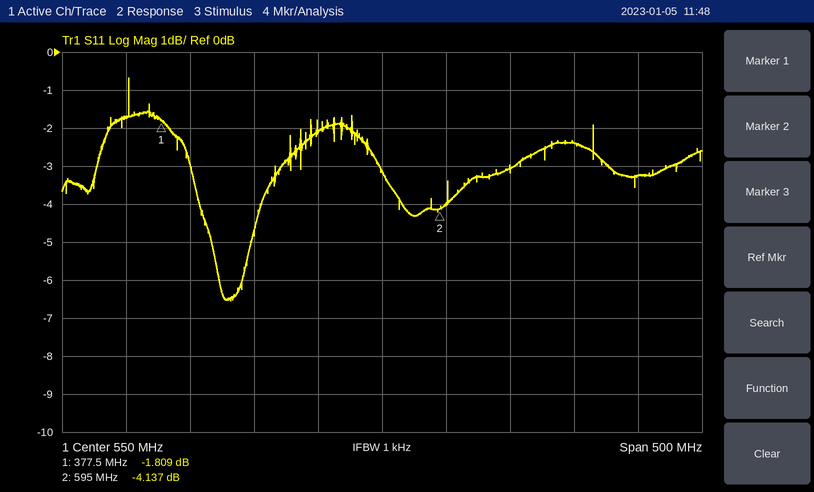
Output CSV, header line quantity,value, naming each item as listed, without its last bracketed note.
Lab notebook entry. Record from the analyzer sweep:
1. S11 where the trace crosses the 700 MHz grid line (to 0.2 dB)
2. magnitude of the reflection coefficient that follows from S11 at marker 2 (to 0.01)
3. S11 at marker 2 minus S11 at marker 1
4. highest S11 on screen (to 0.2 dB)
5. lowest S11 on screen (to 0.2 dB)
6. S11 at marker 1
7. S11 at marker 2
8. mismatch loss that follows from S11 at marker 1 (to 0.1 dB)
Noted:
quantity,value
S11 where the trace crosses the 700 MHz grid line,-2.4 dB
magnitude of the reflection coefficient that follows from S11 at marker 2,0.62
S11 at marker 2 minus S11 at marker 1,-2.328 dB
highest S11 on screen,-0.6 dB
lowest S11 on screen,-6.6 dB
S11 at marker 1,-1.809 dB
S11 at marker 2,-4.137 dB
mismatch loss that follows from S11 at marker 1,4.7 dB
